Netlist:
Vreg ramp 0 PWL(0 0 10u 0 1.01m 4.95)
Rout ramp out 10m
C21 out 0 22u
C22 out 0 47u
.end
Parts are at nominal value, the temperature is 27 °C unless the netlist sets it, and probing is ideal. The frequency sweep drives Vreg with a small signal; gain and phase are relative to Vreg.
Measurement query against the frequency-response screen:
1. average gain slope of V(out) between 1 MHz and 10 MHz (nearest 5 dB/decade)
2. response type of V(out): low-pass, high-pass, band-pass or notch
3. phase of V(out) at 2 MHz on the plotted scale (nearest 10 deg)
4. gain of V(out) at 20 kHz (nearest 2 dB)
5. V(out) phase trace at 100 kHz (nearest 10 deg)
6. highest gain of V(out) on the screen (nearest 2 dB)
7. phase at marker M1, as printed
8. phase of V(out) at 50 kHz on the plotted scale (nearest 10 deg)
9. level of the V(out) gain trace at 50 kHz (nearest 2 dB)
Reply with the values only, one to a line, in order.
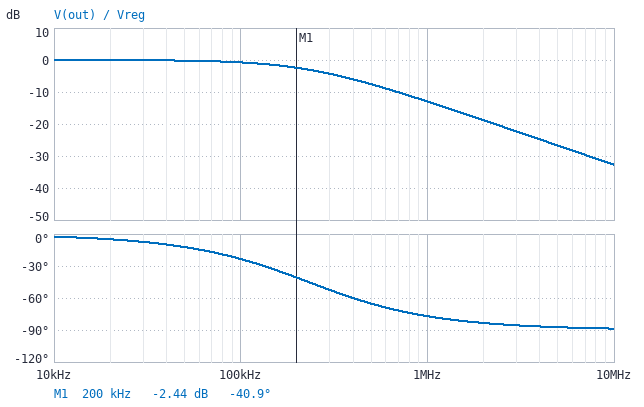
-20 dB/decade
low-pass
-80 deg
0 dB
-20 deg
0 dB
-40.9 deg
-10 deg
0 dB
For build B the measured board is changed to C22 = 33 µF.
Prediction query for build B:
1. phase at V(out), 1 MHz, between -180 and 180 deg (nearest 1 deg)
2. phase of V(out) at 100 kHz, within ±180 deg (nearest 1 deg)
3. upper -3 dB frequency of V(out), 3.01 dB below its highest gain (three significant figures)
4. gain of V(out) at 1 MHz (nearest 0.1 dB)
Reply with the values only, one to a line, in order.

-74 deg
-19 deg
289 kHz
-11.1 dB
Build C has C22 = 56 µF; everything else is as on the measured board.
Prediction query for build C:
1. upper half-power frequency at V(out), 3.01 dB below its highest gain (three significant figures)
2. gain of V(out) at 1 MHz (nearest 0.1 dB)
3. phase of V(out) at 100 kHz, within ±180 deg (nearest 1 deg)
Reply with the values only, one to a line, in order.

204 kHz
-14.0 dB
-26 deg
